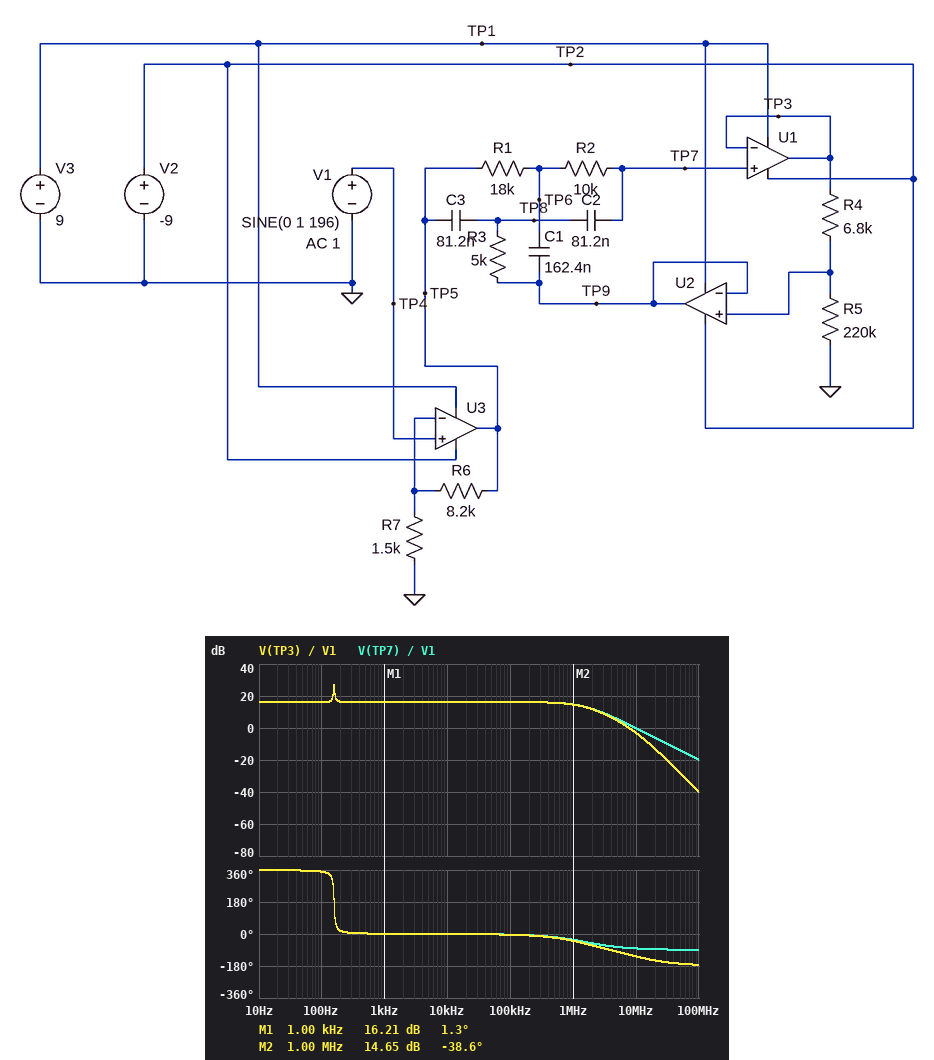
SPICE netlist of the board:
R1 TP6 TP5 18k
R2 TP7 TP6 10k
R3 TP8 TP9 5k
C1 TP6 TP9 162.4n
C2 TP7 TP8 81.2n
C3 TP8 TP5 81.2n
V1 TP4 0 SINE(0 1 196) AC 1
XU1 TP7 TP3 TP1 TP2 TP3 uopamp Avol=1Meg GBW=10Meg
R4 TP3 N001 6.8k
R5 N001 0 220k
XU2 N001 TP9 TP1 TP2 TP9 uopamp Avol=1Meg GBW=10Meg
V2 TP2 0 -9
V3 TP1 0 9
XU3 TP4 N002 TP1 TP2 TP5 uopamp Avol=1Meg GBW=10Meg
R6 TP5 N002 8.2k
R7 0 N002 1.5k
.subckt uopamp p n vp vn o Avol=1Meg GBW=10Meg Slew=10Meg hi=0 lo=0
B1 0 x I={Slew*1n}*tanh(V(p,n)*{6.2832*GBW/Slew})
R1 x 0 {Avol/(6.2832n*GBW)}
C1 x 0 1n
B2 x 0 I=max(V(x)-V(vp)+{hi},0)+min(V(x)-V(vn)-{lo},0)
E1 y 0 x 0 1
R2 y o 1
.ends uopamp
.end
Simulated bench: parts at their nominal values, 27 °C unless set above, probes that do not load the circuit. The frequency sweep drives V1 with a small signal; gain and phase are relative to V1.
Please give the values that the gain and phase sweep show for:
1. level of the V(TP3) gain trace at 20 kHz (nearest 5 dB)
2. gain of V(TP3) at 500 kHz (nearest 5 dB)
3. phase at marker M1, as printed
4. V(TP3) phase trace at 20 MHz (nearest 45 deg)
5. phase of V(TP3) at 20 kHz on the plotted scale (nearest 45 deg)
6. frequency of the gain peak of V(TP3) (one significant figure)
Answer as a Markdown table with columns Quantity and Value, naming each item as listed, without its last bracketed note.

| Quantity | Value |
|---|---|
| level of the V(TP3) gain trace at 20 kHz | 15 dB |
| gain of V(TP3) at 500 kHz | 15 dB |
| phase at marker M1, as printed | 1.3 deg |
| V(TP3) phase trace at 20 MHz | -135 deg |
| phase of V(TP3) at 20 kHz on the plotted scale | 0 deg |
| frequency of the gain peak of V(TP3) | 200 Hz |
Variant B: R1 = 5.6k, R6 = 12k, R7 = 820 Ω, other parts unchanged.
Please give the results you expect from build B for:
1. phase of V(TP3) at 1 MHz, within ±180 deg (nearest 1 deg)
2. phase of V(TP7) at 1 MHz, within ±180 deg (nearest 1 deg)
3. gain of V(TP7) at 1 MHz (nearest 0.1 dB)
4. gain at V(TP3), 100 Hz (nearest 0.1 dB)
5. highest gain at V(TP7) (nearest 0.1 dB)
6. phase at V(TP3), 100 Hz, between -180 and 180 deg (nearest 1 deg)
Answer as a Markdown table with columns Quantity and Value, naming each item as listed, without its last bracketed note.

| Quantity | Value |
|---|---|
| phase of V(TP3) at 1 MHz, within ±180 deg | -63 deg |
| phase of V(TP7) at 1 MHz, within ±180 deg | -57 deg |
| gain of V(TP7) at 1 MHz | 18.5 dB |
| gain at V(TP3), 100 Hz | 23.8 dB |
| highest gain at V(TP7) | 23.9 dB |
| phase at V(TP3), 100 Hz, between -180 and 180 deg | -3 deg |
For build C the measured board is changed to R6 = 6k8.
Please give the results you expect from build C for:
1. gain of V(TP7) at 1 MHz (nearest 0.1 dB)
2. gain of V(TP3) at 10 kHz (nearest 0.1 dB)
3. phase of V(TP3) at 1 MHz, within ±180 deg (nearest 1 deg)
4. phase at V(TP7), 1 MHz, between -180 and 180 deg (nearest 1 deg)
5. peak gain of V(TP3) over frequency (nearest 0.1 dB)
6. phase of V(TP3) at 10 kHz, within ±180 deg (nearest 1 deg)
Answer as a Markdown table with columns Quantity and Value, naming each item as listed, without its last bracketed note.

| Quantity | Value |
|---|---|
| gain of V(TP7) at 1 MHz | 13.7 dB |
| gain of V(TP3) at 10 kHz | 14.9 dB |
| phase of V(TP3) at 1 MHz, within ±180 deg | -35 deg |
| phase at V(TP7), 1 MHz, between -180 and 180 deg | -29 deg |
| peak gain of V(TP3) over frequency | 25.6 dB |
| phase of V(TP3) at 10 kHz, within ±180 deg | 0 deg |
